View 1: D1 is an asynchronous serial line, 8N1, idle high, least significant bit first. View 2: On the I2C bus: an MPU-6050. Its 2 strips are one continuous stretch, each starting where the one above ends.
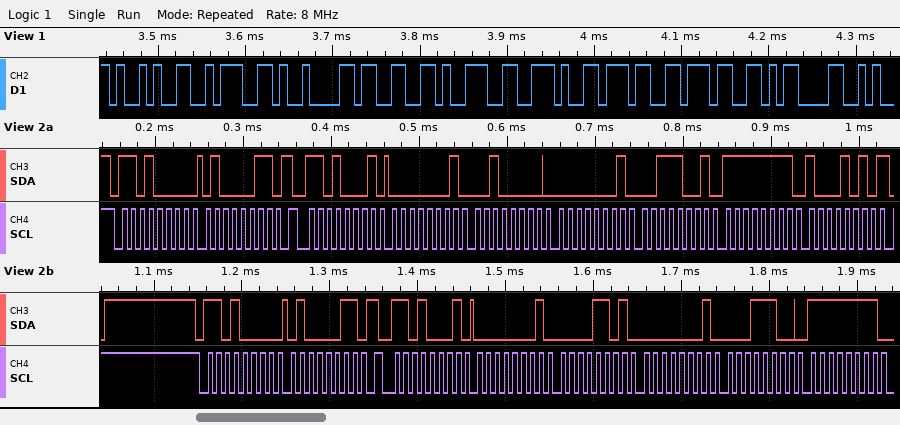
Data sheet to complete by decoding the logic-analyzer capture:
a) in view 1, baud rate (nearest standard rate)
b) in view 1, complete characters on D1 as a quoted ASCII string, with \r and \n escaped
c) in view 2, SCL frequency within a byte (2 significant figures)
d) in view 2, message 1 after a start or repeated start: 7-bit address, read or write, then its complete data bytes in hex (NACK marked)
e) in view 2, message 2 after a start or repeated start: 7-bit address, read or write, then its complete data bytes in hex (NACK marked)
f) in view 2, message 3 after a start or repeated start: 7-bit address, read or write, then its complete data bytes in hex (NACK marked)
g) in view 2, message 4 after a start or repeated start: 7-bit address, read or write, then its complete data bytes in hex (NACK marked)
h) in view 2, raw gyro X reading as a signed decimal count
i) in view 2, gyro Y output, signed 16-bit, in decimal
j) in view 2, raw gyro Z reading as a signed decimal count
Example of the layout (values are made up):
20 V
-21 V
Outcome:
115200 baud
"):\t39.77\r"
100 kHz
0x68 write: 43
0x68 read: 01 20 01 39 FF 8A NACK
0x68 write: 43
0x68 read: 01 0D 01 1C FF
288
313
-118
